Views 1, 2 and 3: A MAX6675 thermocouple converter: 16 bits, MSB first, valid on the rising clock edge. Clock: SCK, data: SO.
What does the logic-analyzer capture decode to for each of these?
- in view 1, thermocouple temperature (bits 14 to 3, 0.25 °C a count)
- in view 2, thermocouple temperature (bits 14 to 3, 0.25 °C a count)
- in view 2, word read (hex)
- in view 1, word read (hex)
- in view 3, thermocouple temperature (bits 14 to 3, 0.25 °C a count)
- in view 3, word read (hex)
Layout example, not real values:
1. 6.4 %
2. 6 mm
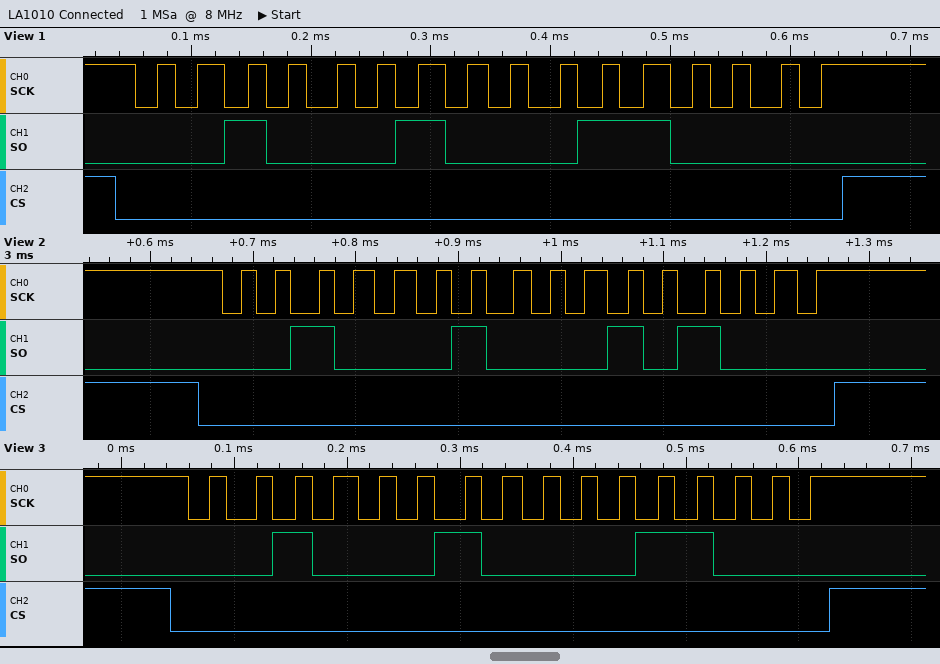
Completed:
1. 273.50 °C
2. 273.25 °C
3. 0x2228
4. 0x2230
5. 272.75 °C
6. 0x2218
